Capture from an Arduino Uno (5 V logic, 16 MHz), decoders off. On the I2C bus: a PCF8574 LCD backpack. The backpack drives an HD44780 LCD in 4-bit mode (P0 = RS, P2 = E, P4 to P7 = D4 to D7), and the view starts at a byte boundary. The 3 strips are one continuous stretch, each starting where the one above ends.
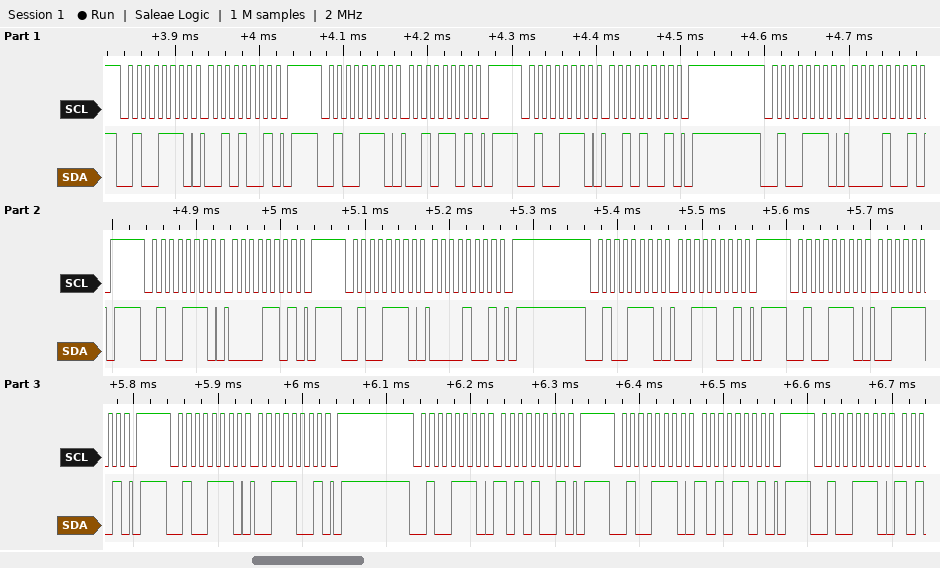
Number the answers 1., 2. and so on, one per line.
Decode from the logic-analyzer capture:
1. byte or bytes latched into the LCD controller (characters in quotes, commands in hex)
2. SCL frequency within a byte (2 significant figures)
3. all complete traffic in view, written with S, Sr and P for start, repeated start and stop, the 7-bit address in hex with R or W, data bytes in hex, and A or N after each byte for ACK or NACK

1. ' '
2. 100 kHz
3. S 27W A 29 A P S 27W A 2D A P S 27W A 29 A P S 27W A 09 A P S 27W A 0D A P S 27W A 09 A P S 27W A 39 A P S 27W A 3D A P S 27W A 39 A P S 27W A A9 A P S 27W A AD A P S 27W A
